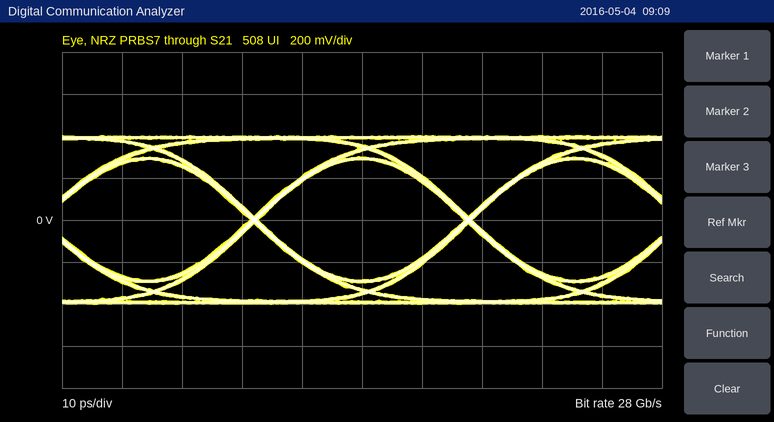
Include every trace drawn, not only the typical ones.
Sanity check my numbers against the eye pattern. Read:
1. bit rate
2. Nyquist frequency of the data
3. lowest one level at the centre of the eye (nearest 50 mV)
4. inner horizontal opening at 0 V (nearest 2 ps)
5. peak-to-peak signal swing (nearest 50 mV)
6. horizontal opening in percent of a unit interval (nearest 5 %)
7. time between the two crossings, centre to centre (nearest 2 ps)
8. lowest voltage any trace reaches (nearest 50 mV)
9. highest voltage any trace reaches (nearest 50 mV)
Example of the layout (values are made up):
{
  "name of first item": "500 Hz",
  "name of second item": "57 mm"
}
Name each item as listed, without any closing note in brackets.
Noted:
{
  "bit rate": "28 Gb/s",
  "Nyquist frequency of the data": "14 GHz",
  "lowest one level at the centre of the eye": "300 mV",
  "inner horizontal opening at 0 V": "34 ps",
  "peak-to-peak signal swing": "800 mV",
  "horizontal opening in percent of a unit interval": "95 %",
  "time between the two crossings, centre to centre": "36 ps",
  "lowest voltage any trace reaches": "-400 mV",
  "highest voltage any trace reaches": "400 mV"
}
